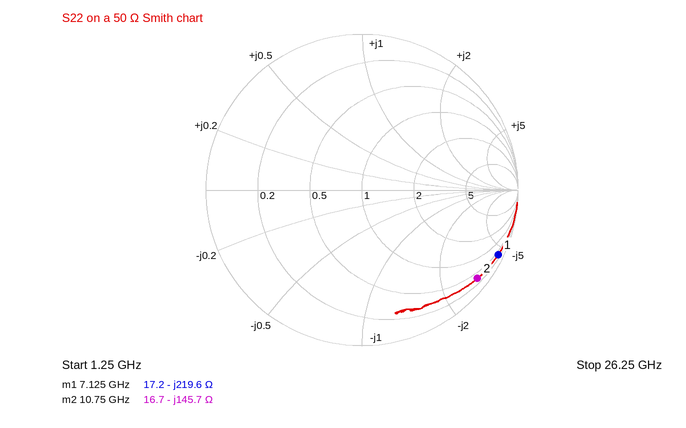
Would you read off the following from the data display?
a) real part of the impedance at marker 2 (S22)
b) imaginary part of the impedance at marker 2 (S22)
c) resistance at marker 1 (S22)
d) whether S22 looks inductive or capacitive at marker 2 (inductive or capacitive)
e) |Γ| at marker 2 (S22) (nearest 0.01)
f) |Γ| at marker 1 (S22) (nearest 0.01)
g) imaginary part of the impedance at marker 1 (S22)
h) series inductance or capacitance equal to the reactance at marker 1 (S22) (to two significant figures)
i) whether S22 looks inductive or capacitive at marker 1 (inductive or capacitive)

16.7 Ω
-145.7 Ω
17.2 Ω
capacitive
0.93
0.97
-219.6 Ω
100 fF
capacitive
